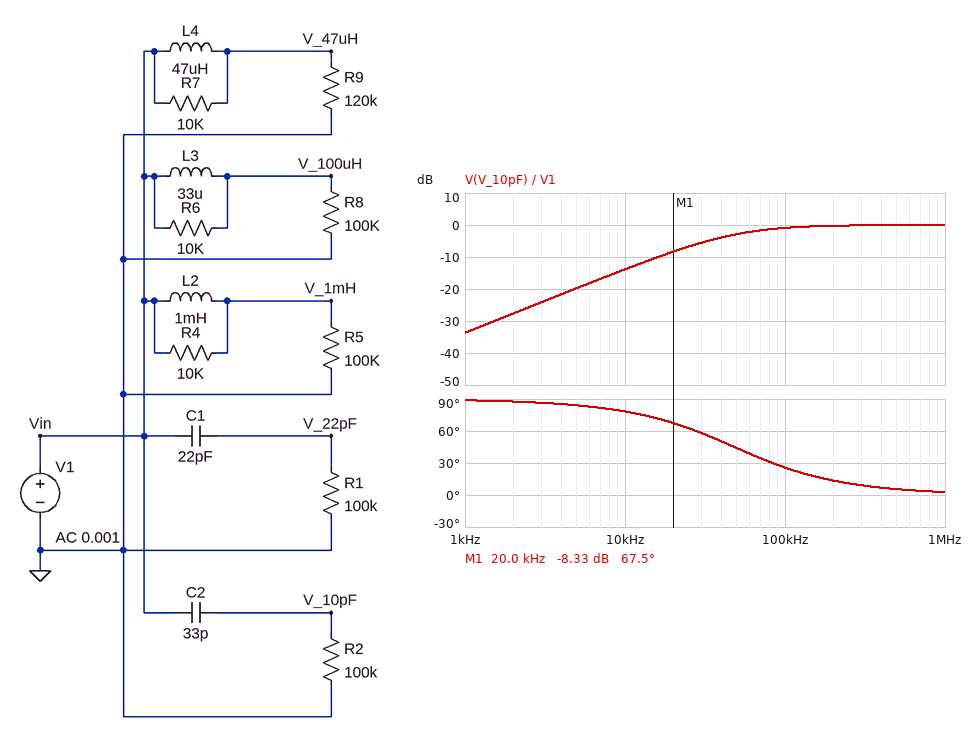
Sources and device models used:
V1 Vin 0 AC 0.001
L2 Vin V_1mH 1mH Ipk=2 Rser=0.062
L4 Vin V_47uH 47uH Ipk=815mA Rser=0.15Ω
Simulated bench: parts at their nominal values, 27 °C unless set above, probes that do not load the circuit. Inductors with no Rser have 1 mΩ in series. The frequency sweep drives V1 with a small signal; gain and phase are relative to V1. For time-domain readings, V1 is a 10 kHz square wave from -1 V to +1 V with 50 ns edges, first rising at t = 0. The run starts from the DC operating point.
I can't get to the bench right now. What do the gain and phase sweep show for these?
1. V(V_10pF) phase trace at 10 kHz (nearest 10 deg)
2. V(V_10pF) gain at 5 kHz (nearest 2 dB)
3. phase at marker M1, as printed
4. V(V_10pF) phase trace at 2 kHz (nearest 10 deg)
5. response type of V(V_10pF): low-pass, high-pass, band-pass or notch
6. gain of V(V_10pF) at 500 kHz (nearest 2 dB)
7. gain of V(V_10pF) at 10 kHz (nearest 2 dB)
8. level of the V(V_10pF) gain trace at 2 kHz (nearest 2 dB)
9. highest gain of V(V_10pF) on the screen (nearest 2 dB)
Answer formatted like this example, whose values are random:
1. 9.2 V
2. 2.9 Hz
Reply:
1. 80 deg
2. -20 dB
3. 67.5 deg
4. 90 deg
5. high-pass
6. 0 dB
7. -14 dB
8. -28 dB
9. 0 dB
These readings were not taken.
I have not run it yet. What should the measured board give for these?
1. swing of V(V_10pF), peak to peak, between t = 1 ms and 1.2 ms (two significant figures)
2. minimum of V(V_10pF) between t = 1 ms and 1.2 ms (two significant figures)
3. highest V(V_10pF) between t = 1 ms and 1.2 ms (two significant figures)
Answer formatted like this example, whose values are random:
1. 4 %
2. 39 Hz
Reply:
1. 4.0 V
2. -2.0 V
3. 2.0 V
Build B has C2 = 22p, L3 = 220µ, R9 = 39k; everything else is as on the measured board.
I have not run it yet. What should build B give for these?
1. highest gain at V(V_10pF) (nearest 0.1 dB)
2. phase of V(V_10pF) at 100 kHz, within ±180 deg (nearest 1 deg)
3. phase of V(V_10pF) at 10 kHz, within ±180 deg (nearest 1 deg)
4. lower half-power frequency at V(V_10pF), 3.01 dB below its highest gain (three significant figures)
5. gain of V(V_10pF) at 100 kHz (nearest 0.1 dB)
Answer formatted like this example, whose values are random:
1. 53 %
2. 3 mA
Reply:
1. 0 dB
2. 36 deg
3. 82 deg
4. 72.3 kHz
5. -1.8 dB
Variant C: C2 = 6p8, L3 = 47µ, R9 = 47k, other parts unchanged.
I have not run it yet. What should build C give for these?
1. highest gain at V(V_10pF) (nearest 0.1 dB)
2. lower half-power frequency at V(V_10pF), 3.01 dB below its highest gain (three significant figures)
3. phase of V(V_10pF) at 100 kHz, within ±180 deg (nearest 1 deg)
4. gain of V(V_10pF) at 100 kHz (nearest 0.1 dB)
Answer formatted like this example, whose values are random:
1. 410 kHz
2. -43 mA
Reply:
1. 0 dB
2. 234 kHz
3. 67 deg
4. -8.1 dB
